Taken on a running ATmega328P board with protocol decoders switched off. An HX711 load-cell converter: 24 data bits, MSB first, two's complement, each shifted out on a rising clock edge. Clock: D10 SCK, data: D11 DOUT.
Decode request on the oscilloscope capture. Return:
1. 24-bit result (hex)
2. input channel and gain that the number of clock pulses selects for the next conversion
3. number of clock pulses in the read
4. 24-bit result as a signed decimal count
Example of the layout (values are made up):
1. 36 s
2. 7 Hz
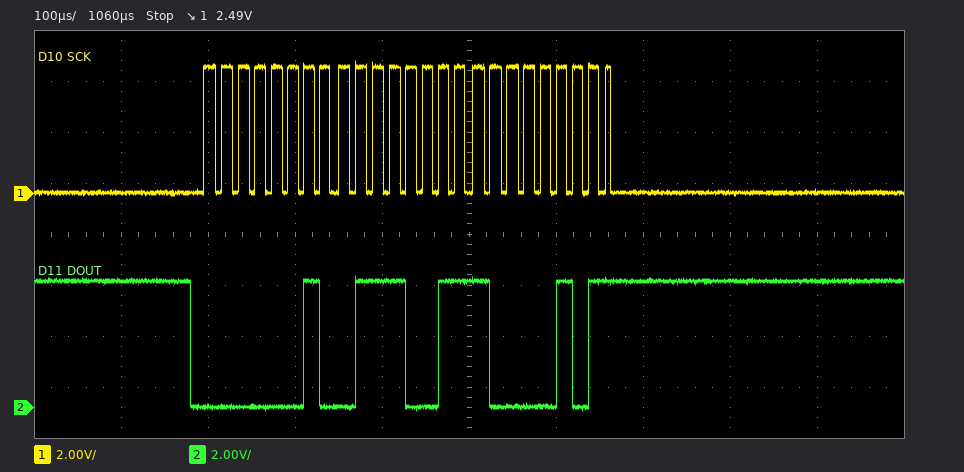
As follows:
1. 0x027385
2. channel A, gain 128
3. 25
4. 160645
